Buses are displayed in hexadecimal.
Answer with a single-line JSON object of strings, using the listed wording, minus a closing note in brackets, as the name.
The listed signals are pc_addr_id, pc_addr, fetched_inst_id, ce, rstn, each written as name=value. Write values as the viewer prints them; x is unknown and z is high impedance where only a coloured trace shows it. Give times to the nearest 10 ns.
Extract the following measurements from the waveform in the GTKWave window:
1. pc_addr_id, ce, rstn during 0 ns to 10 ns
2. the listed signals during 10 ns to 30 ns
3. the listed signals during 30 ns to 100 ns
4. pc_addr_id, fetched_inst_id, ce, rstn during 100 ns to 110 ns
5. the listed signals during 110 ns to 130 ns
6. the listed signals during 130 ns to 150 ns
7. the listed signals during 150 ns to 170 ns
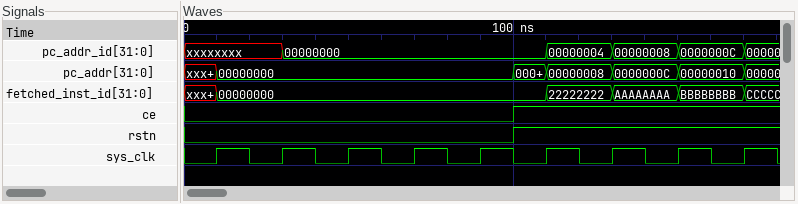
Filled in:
{"pc_addr_id, ce, rstn during 0 ns to 10 ns": "pc_addr_id=xxxxxxxx, ce=0, rstn=0", "the listed signals during 10 ns to 30 ns": "pc_addr_id=xxxxxxxx, pc_addr=00000000, fetched_inst_id=00000000, ce=0, rstn=0", "the listed signals during 30 ns to 100 ns": "pc_addr_id=00000000, pc_addr=00000000, fetched_inst_id=00000000, ce=0, rstn=0", "pc_addr_id, fetched_inst_id, ce, rstn during 100 ns to 110 ns": "pc_addr_id=00000000, fetched_inst_id=00000000, ce=1, rstn=1", "the listed signals during 110 ns to 130 ns": "pc_addr_id=00000004, pc_addr=00000008, fetched_inst_id=22222222, ce=1, rstn=1", "the listed signals during 130 ns to 150 ns": "pc_addr_id=00000008, pc_addr=0000000C, fetched_inst_id=AAAAAAAA, ce=1, rstn=1", "the listed signals during 150 ns to 170 ns": "pc_addr_id=0000000C, pc_addr=00000010, fetched_inst_id=BBBBBBBB, ce=1, rstn=1"}
